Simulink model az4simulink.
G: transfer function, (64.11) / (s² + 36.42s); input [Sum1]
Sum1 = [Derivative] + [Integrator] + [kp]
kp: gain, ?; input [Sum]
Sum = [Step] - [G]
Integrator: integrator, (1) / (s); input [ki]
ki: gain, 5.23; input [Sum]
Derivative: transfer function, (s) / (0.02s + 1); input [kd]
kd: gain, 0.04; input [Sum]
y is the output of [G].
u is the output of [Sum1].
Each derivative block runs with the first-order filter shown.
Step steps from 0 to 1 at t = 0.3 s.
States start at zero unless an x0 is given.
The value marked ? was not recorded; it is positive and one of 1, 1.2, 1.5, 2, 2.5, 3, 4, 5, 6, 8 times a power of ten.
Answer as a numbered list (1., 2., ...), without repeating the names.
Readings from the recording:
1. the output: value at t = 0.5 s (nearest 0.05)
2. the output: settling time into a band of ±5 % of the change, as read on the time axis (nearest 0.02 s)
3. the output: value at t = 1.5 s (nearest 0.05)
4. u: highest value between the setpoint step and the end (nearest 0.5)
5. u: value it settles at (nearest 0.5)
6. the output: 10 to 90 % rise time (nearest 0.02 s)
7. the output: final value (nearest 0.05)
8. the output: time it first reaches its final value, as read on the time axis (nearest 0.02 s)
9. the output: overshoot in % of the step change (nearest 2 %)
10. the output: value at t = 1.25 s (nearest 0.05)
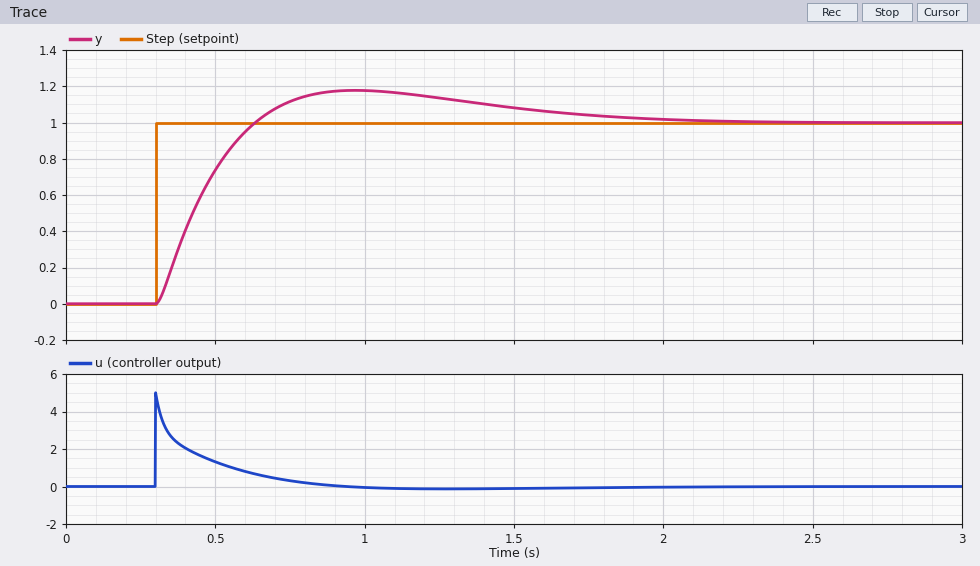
1. 0.75
2. 1.68 s
3. 1.10
4. 5.0
5. 0.0
6. 0.24 s
7. 1.00
8. 0.64 s
9. 18 %
10. 1.15
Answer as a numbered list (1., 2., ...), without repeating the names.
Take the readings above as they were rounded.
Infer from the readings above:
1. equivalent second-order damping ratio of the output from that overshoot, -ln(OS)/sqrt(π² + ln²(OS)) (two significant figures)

1. 0.48
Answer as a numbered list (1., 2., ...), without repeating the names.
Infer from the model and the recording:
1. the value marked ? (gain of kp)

1. 3
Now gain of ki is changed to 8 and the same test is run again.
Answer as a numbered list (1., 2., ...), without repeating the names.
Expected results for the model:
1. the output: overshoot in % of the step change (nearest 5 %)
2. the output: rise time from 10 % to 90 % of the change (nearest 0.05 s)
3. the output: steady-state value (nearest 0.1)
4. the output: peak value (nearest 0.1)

1. 25 %
2. 0.20 s
3. 1.0
4. 1.2
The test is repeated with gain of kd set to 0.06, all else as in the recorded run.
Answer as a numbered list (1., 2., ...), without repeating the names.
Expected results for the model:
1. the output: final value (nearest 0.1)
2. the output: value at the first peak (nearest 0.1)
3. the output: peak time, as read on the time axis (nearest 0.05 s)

1. 1.0
2. 1.2
3. 1.00 s
